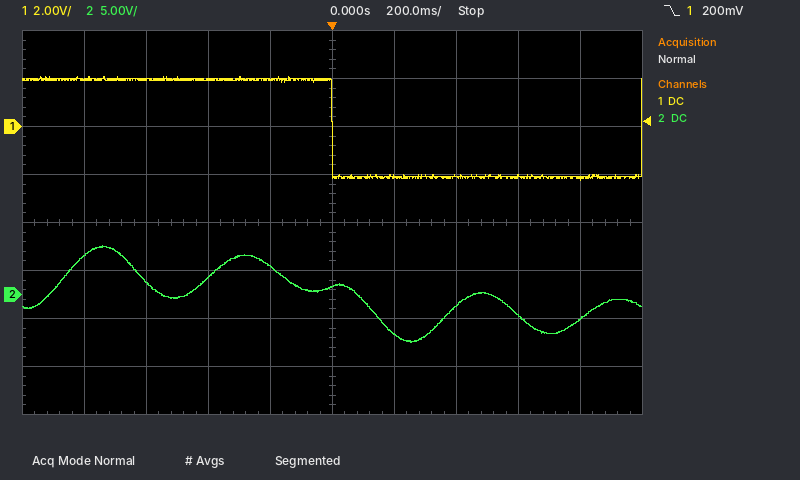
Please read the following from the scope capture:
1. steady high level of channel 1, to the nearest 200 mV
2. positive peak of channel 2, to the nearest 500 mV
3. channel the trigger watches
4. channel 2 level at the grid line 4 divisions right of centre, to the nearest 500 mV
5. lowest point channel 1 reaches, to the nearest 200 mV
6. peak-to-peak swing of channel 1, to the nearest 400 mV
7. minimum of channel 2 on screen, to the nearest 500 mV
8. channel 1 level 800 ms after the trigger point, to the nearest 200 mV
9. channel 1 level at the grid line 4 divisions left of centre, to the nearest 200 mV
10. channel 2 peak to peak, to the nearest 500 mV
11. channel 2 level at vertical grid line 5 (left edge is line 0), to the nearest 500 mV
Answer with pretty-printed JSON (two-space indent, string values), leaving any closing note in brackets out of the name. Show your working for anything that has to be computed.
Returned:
{
  "steady high level of channel 1, to the nearest 200 mV": "2.0 V",
  "positive peak of channel 2, to the nearest 500 mV": "5.0 V",
  "channel the trigger watches": "channel 1",
  "channel 2 level at the grid line 4 divisions right of centre, to the nearest 500 mV": "-2.5 V",
  "lowest point channel 1 reaches, to the nearest 200 mV": "-2.2 V",
  "peak-to-peak swing of channel 1, to the nearest 400 mV": "4.4 V",
  "minimum of channel 2 on screen, to the nearest 500 mV": "-5.0 V",
  "channel 1 level 800 ms after the trigger point, to the nearest 200 mV": "-2.2 V",
  "channel 1 level at the grid line 4 divisions left of centre, to the nearest 200 mV": "2.0 V",
  "channel 2 peak to peak, to the nearest 500 mV": "5.0 V − (-5.0 V) = 10.0 V",
  "channel 2 level at vertical grid line 5 (left edge is line 0), to the nearest 500 mV": "1.0 V"
}
